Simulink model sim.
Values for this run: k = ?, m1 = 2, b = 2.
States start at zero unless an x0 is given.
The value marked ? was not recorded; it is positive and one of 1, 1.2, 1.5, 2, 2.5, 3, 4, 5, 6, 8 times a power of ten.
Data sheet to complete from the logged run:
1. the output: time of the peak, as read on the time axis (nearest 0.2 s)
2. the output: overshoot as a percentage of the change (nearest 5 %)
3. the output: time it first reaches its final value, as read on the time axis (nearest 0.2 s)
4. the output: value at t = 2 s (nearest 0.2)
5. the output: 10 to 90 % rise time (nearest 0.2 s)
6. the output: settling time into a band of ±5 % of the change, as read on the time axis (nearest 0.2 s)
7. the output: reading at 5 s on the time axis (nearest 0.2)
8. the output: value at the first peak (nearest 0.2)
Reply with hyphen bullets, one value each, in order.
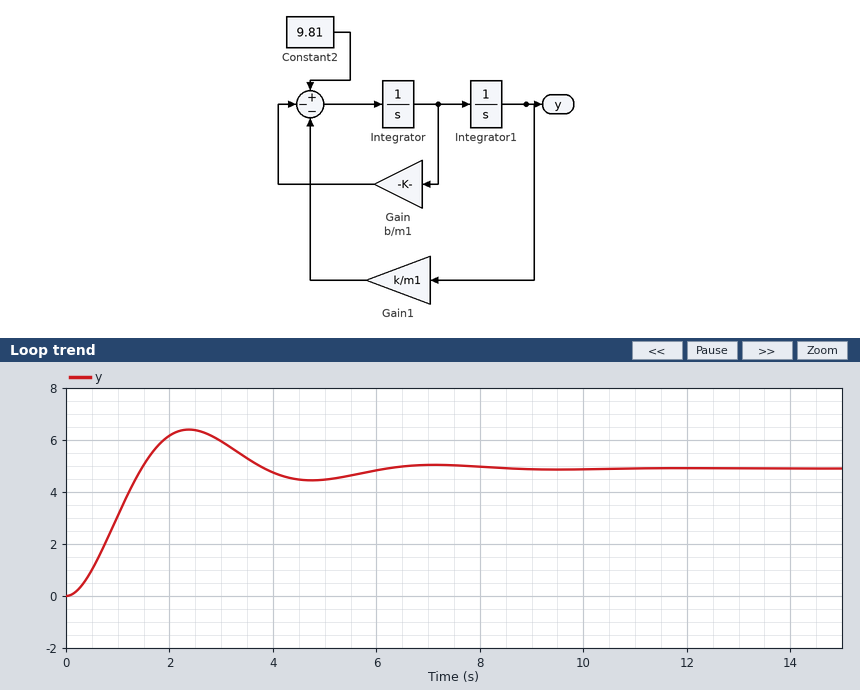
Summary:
- 2.4 s
- 30 %
- 1.4 s
- 6.2
- 1.0 s
- 5.6 s
- 4.4
- 6.4
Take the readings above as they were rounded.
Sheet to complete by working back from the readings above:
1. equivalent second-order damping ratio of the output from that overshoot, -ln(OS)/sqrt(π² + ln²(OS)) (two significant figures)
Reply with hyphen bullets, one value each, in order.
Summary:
- 0.36
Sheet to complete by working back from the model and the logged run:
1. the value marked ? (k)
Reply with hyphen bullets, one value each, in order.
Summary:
- 4
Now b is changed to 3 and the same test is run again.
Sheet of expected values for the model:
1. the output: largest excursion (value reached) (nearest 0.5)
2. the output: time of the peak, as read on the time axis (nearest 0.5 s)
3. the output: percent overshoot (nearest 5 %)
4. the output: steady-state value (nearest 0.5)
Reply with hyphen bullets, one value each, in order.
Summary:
- 5.5
- 2.5 s
- 15 %
- 5.0
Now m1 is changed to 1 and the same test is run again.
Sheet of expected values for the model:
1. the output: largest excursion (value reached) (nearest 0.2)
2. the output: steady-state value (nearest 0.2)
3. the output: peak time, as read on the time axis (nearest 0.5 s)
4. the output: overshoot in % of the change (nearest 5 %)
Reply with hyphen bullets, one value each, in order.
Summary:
- 2.8
- 2.4
- 2.0 s
- 15 %
